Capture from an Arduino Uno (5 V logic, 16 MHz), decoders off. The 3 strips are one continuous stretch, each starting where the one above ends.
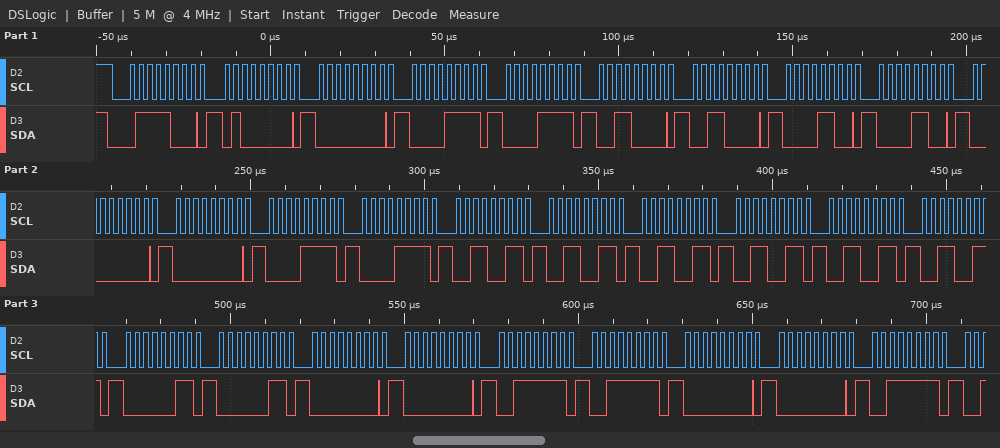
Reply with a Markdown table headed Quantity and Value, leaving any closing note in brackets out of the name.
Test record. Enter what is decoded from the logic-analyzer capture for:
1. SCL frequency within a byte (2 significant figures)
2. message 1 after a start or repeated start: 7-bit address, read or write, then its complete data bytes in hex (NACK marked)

| Quantity | Value |
|---|---|
| SCL frequency within a byte | 400 kHz |
| message 1 after a start or repeated start: 7-bit address, read or write, then its complete data bytes in hex | 0x3C write: 40 00 0F 0F 30 30 0C 0C 00 00 0F 0F 33 33 33 33 33 33 03 03 00 00 3F 3F 00 00 3F |
